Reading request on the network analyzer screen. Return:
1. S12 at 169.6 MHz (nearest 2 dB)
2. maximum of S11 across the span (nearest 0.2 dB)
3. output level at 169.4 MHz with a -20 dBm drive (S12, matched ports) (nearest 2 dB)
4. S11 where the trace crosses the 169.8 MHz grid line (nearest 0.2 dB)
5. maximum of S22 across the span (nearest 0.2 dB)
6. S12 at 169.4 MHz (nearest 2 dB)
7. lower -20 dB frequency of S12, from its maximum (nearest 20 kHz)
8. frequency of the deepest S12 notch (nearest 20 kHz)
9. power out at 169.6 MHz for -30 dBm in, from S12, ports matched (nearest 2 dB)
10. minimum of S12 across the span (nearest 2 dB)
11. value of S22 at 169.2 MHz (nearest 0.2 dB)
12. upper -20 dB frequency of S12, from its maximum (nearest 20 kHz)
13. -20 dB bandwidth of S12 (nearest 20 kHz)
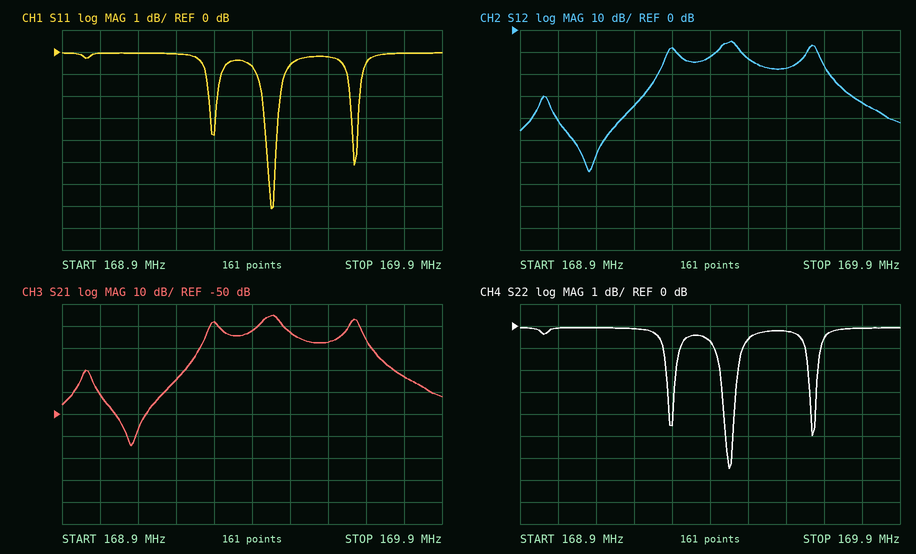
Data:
-18 dB
0.0 dB
-32 dBm
0.0 dB
0.0 dB
-12 dB
169.24 MHz
169.08 MHz
-48 dBm
-64 dB
-0.2 dB
169.74 MHz
500 kHz
